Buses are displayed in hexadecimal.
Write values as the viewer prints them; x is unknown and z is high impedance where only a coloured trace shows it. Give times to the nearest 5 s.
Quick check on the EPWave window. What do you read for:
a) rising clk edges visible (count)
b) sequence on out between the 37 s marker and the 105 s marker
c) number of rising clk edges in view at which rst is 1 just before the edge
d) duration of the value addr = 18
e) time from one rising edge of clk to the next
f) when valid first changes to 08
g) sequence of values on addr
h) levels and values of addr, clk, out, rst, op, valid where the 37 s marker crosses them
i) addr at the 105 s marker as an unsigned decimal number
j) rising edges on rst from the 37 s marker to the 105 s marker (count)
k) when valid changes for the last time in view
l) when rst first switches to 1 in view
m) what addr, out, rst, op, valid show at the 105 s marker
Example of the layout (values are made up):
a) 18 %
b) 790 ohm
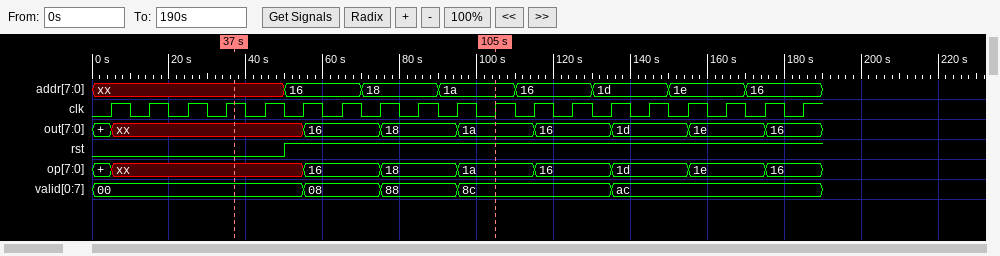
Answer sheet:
a) 19
b) xx, 16, 18, 1a
c) 14
d) 20 s
e) 10 s
f) 55 s
g) xx, 16, 18, 1a, 16, 1d, 1e, 16
h) addr=xx, clk=1, out=xx, rst=0, op=xx, valid=00
i) 26
j) 1
k) 135 s
l) 50 s
m) addr=1a, out=1a, rst=1, op=1a, valid=8c
